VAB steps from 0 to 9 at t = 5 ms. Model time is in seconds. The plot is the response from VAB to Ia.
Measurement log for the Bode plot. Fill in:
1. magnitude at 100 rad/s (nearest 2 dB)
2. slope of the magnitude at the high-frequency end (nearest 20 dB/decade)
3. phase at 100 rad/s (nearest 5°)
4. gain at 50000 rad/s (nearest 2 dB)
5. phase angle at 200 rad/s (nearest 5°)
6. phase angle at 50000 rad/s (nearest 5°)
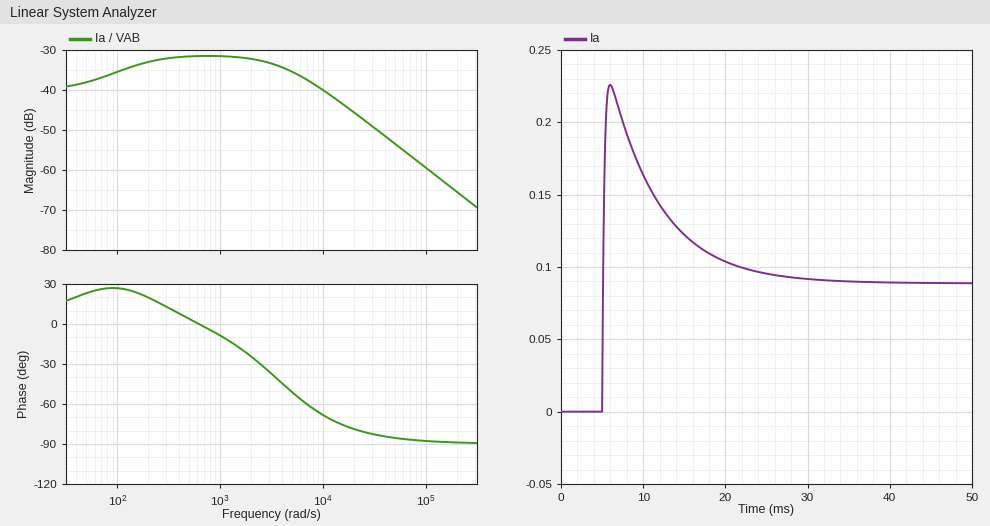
-36 dB
-20 dB/decade
25°
-54 dB
20°
-85°
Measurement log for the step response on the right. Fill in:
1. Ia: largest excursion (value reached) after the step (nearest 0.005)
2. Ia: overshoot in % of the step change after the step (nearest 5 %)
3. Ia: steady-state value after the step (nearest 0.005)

0.225
155 %
0.090
